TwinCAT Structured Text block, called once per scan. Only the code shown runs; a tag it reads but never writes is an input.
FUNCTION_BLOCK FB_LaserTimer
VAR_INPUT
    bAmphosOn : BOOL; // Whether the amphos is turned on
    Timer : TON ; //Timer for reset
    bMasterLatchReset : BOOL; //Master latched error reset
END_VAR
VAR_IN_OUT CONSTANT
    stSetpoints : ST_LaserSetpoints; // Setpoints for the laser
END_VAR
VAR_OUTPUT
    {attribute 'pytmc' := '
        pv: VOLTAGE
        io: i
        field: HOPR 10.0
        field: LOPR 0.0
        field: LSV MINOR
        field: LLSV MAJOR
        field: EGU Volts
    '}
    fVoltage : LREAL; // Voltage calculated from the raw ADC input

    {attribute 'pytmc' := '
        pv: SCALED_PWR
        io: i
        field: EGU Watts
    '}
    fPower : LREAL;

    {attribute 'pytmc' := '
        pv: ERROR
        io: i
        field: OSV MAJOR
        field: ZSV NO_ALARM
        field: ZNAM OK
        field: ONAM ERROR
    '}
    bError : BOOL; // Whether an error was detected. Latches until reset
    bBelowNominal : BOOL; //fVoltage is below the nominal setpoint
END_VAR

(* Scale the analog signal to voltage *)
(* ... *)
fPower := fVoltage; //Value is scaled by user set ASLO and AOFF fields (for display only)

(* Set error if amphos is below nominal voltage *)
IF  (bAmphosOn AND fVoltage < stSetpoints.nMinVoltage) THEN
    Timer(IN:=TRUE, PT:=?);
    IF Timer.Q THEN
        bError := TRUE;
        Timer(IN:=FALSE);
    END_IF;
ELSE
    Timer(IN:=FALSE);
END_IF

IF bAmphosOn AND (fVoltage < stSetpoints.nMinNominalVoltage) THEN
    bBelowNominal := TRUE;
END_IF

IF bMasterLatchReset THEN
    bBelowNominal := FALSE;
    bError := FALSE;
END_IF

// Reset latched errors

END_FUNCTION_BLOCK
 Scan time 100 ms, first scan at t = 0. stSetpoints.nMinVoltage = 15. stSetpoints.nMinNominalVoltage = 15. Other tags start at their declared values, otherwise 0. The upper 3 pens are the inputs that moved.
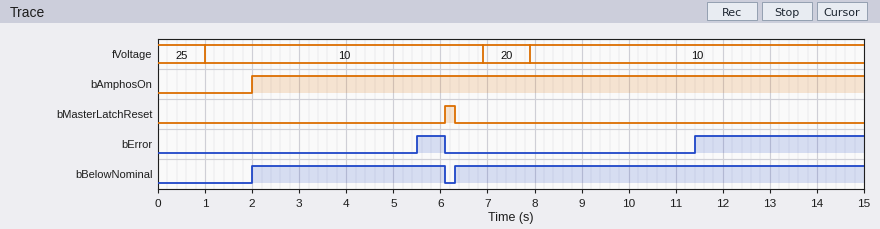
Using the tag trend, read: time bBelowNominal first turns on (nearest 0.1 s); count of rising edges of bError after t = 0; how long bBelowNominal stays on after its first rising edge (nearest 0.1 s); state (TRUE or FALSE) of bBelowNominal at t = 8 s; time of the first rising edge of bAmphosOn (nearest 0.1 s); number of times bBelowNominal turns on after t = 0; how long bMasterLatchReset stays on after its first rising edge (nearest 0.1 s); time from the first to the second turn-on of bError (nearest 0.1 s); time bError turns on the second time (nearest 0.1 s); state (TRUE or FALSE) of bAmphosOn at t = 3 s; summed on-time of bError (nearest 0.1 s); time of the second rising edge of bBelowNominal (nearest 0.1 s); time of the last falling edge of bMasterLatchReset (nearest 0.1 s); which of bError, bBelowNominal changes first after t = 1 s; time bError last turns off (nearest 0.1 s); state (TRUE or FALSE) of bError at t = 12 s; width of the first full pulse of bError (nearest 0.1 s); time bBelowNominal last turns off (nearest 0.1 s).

2.0 s
2
4.1 s
TRUE
2.0 s
2
0.2 s
5.9 s
11.4 s
TRUE
4.2 s
6.3 s
6.3 s
bBelowNominal
6.1 s
TRUE
0.6 s
6.1 s
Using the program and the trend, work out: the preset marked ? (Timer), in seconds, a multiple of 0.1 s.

3.5 s
